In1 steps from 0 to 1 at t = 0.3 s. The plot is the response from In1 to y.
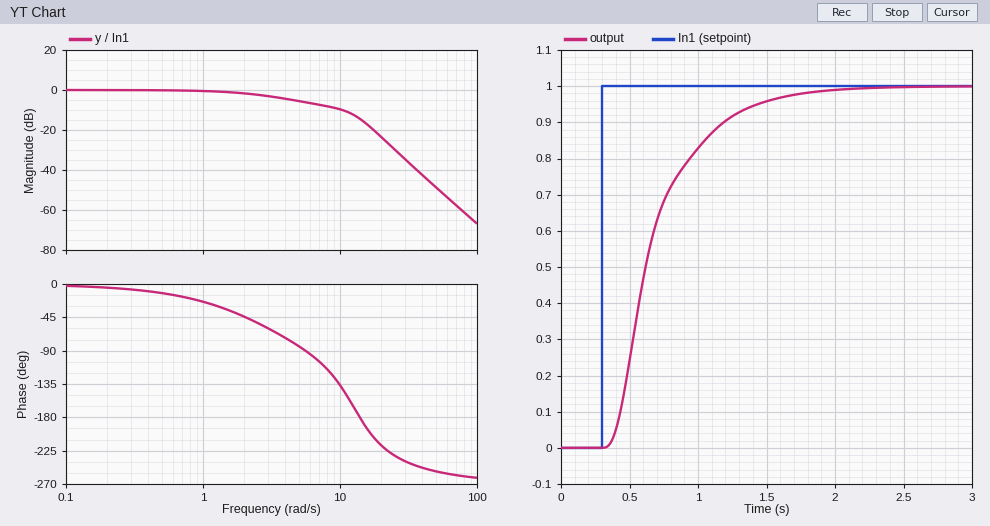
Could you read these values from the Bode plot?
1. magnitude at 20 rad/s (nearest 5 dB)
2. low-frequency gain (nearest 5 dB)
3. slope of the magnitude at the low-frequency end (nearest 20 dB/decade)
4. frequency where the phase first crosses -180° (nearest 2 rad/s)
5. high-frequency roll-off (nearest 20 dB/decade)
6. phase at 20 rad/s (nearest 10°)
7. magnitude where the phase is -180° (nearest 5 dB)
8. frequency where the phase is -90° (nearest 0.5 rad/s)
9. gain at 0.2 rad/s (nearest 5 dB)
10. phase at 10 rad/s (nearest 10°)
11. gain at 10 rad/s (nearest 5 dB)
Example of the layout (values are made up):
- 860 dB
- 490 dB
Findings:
- -25 dB
- 0 dB
- 0 dB/decade
- 14 rad/s
- -60 dB/decade
- -220°
- -15 dB
- 5.5 rad/s
- 0 dB
- -140°
- -10 dB
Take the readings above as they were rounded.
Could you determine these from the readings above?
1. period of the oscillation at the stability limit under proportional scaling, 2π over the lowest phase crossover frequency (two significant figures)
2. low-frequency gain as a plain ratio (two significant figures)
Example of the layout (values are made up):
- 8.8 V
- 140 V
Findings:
- 0.45 s
- 1.0
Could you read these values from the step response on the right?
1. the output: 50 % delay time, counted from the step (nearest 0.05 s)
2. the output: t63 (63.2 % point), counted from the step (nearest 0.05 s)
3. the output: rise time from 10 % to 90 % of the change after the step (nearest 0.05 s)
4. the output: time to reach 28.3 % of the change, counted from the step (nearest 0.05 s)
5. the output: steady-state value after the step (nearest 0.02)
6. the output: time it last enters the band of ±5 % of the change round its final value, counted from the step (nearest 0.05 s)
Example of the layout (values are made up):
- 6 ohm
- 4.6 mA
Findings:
- 0.30 s
- 0.40 s
- 0.75 s
- 0.20 s
- 1.00
- 1.15 s
